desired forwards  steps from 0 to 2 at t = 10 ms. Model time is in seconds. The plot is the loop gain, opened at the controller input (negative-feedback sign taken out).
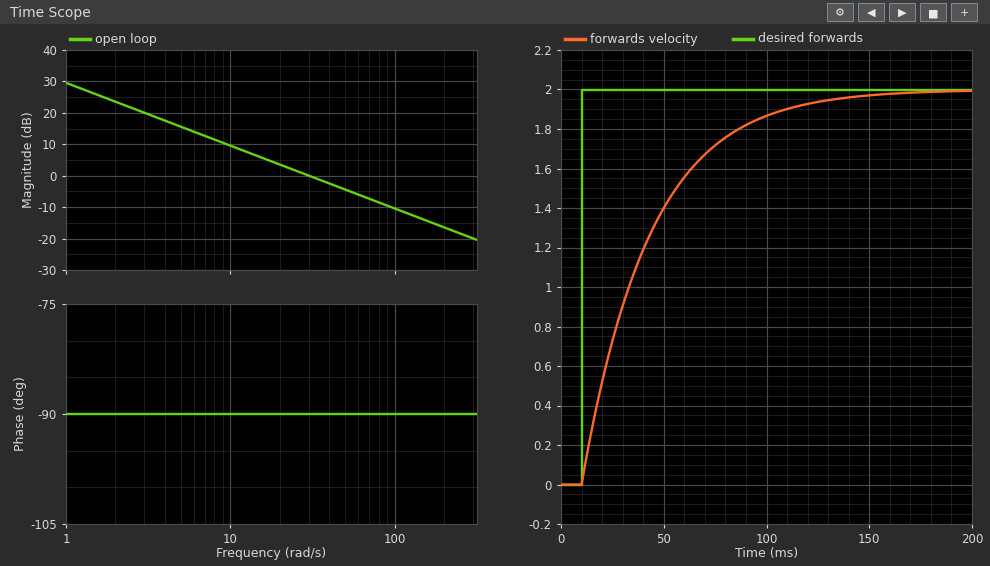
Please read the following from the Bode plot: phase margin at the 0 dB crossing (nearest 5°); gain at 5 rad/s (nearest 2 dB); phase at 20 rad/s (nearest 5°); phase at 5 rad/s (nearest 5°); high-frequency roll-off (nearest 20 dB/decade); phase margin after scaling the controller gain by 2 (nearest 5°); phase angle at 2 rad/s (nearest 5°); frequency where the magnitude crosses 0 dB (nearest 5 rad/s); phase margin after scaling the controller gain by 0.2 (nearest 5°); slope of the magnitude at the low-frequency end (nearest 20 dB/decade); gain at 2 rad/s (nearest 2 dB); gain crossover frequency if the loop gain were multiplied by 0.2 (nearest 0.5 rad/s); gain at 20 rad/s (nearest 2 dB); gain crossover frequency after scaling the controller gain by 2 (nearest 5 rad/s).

90°
16 dB
-90°
-90°
-20 dB/decade
90°
-90°
30 rad/s
90°
-20 dB/decade
24 dB
6.0 rad/s
4 dB
60 rad/s
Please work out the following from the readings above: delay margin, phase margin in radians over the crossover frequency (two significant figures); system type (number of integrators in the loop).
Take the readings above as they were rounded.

0.052 s
1
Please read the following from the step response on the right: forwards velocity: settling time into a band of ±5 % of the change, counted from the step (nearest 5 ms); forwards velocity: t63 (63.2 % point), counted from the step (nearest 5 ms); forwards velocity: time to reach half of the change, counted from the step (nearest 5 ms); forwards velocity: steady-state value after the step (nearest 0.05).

100 ms
35 ms
25 ms
2.00
